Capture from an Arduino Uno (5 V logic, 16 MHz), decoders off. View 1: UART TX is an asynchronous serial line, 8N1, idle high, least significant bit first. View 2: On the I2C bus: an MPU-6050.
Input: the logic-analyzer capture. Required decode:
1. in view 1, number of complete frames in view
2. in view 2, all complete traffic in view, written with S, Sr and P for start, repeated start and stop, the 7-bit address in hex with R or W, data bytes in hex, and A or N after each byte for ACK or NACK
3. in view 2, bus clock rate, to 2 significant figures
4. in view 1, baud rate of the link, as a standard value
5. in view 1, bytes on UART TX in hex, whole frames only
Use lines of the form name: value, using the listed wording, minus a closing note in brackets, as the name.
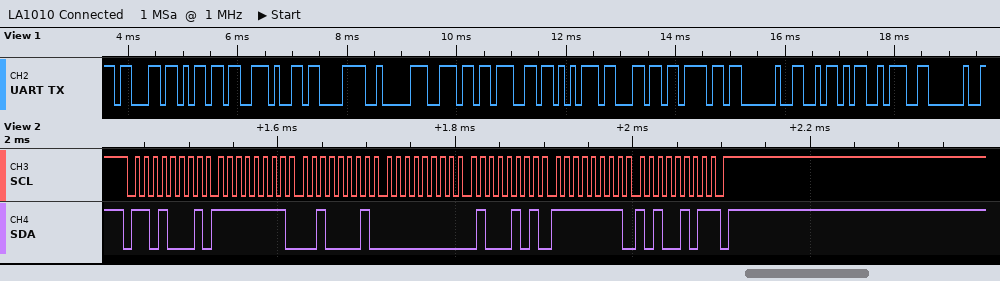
in view 1, number of complete frames in view: 14
in view 2, all complete traffic in view, written with S, Sr and P for start, repeated start and stop, the 7-bit address in hex with R or W, data bytes in hex, and A or N after each byte for ACK or NACK: S 68R A FF A 21 A 00 A 45 A FF A A5 N P
in view 2, bus clock rate, to 2 significant figures: 100 kHz
in view 1, baud rate of the link, as a standard value: 9600 baud
in view 1, bytes on UART TX in hex, whole frames only: 0x63 0x6D 0x2E 0xC3 0x82 0x6E 0x67 0x75 0x6C 0x6F 0x20 0x5A 0x3A 0x20
